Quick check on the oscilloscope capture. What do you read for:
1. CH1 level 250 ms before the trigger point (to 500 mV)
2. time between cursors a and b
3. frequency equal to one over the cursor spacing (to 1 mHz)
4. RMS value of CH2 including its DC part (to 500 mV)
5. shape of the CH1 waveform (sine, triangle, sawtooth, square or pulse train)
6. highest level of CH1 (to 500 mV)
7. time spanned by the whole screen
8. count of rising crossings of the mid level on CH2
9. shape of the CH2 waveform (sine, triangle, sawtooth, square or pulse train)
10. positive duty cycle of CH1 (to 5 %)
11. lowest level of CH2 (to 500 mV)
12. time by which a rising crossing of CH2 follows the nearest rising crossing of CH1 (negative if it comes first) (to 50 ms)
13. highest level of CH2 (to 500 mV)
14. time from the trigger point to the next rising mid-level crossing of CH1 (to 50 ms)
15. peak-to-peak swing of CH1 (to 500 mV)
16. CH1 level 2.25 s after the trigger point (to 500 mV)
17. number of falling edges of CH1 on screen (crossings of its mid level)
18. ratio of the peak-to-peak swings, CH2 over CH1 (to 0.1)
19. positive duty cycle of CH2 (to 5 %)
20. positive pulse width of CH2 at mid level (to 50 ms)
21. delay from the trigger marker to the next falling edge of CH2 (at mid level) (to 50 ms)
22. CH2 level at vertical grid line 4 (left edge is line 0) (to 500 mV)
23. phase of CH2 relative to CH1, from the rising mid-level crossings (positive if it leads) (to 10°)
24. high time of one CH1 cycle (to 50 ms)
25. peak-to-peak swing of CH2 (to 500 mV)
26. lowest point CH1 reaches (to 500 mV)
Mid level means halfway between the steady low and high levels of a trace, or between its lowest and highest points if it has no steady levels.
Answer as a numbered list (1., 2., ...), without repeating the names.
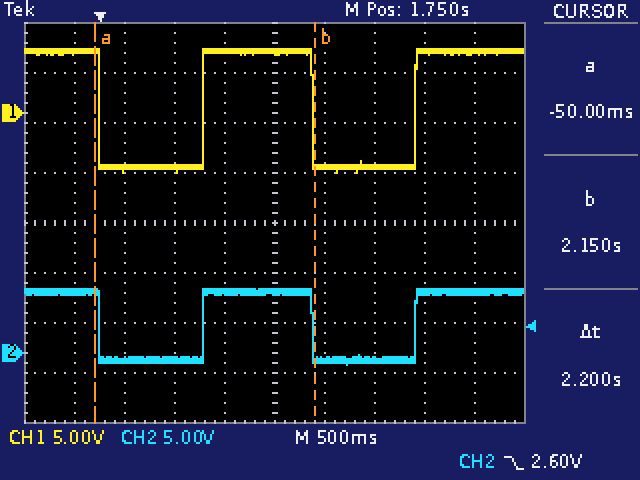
1. 6.0 V
2. 2.2 s
3. 455 mHz
4. 4.5 V
5. square
6. 6.5 V
7. 5 s
8. 2
9. square
10. 50 %
11. -1.0 V
12. 0 ms
13. 6.5 V
14. 1.05 s
15. 12.5 V
16. -5.5 V
17. 2
18. 0.6
19. 50 %
20. 1.10 s
21. 2.15 s
22. 6.0 V
23. 0°
24. 1.10 s
25. 7.5 V
26. -6.0 V
